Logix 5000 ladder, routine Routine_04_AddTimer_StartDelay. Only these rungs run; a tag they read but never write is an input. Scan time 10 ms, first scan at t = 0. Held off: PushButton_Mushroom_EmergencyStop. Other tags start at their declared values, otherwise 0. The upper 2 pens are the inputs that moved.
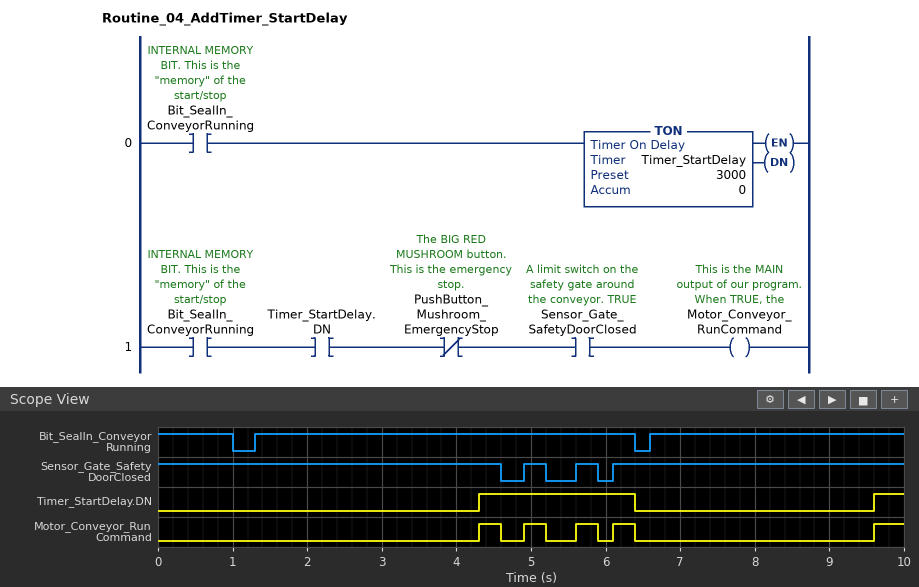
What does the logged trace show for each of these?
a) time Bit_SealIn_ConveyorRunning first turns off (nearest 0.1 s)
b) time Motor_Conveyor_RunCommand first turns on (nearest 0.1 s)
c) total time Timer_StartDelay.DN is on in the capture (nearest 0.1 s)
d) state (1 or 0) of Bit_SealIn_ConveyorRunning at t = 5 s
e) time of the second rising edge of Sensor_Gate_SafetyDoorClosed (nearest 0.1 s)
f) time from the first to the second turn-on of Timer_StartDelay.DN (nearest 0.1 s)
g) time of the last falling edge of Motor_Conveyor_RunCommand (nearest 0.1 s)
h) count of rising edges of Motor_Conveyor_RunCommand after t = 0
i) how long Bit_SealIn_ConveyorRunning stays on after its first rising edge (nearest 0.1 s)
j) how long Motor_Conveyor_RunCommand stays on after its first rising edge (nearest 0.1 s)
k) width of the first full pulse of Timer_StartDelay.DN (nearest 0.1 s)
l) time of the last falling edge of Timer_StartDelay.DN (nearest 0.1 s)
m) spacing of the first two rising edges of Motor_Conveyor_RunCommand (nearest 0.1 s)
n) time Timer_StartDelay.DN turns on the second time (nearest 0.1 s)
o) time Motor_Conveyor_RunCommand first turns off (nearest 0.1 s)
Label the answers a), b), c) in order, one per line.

a) 1.0 s
b) 4.3 s
c) 2.5 s
d) 1
e) 5.6 s
f) 5.3 s
g) 6.4 s
h) 5
i) 5.1 s
j) 0.3 s
k) 2.1 s
l) 6.4 s
m) 0.6 s
n) 9.6 s
o) 4.6 s
